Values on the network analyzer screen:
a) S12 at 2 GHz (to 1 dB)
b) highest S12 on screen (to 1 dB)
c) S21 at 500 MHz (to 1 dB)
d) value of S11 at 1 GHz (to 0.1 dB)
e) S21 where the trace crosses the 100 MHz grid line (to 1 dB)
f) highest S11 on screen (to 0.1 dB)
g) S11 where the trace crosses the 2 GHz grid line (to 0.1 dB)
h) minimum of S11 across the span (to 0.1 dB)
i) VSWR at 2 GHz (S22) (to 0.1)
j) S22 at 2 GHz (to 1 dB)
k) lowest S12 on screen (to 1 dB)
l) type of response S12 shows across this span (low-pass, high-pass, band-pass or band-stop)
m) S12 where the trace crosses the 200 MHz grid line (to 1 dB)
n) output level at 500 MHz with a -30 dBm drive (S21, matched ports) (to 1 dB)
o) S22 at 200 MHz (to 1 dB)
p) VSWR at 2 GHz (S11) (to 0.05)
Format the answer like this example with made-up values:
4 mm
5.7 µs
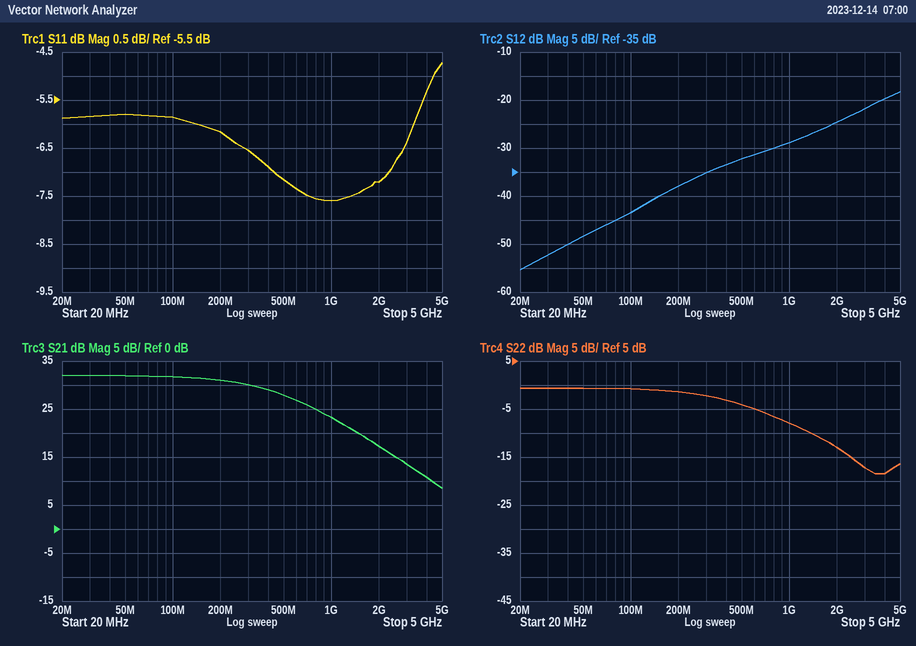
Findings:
-25 dB
-18 dB
28 dB
-7.6 dB
32 dB
-4.7 dB
-7.2 dB
-7.6 dB
1.6
-13 dB
-55 dB
high-pass
-38 dB
-2 dBm
-1 dB
2.55
